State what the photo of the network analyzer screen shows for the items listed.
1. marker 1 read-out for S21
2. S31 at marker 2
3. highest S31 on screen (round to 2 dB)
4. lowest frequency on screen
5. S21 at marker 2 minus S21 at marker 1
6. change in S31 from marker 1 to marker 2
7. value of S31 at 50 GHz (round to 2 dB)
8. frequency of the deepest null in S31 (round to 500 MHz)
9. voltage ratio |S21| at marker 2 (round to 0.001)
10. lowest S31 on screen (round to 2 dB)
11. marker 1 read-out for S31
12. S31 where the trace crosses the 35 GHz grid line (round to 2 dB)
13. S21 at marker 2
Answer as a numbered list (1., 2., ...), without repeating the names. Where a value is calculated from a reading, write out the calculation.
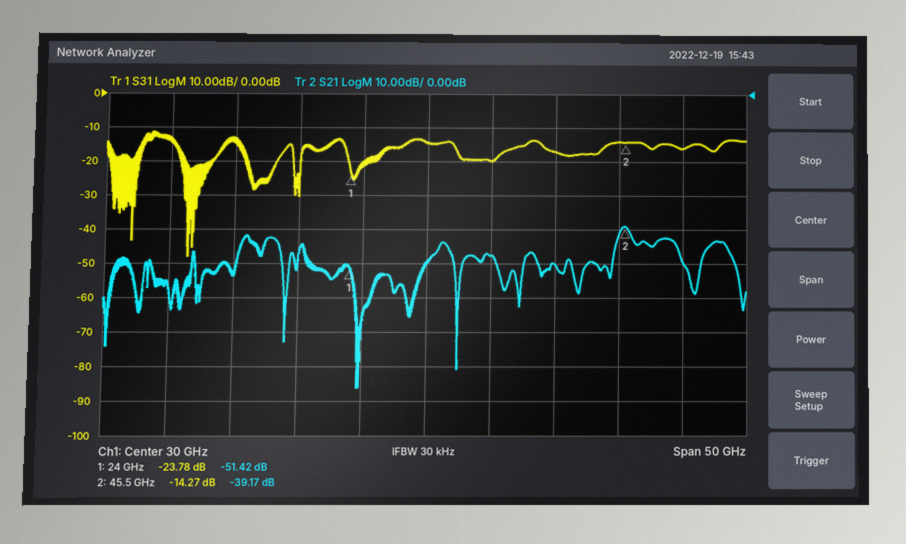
1. -51.42 dB
2. -14.27 dB
3. -12 dB
4. 5 GHz
5. -39.17 − (-51.42) = 12.25 dB
6. -14.27 − (-23.78) = 9.51 dB
7. -16 dB
8. 11.5 GHz
9. 10^(-39.17/20) ≈ 0.011
10. -48 dB
11. -23.78 dB
12. -20 dB
13. -39.17 dB
